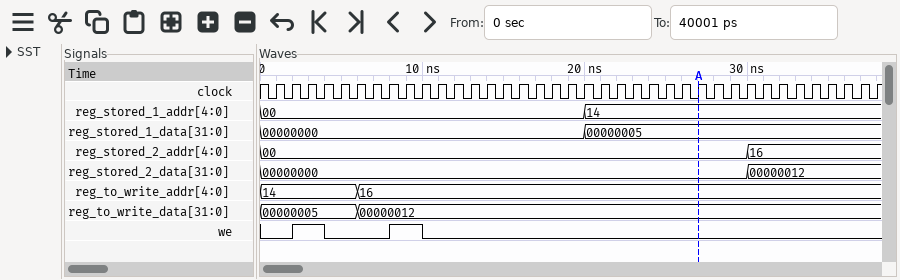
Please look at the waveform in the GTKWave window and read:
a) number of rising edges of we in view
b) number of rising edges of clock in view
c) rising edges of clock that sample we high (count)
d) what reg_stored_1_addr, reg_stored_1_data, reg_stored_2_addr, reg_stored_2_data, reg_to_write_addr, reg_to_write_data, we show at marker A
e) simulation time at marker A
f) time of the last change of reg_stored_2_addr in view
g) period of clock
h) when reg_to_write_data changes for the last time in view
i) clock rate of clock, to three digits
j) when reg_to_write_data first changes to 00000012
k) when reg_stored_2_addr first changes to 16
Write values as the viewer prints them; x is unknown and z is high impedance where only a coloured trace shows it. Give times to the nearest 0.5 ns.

2
38
4
reg_stored_1_addr=14, reg_stored_1_data=00000005, reg_stored_2_addr=00, reg_stored_2_data=00000000, reg_to_write_addr=16, reg_to_write_data=00000012, we=0
27 ns
30 ns
1 ns
6 ns
1.00 GHz
6 ns
30 ns
